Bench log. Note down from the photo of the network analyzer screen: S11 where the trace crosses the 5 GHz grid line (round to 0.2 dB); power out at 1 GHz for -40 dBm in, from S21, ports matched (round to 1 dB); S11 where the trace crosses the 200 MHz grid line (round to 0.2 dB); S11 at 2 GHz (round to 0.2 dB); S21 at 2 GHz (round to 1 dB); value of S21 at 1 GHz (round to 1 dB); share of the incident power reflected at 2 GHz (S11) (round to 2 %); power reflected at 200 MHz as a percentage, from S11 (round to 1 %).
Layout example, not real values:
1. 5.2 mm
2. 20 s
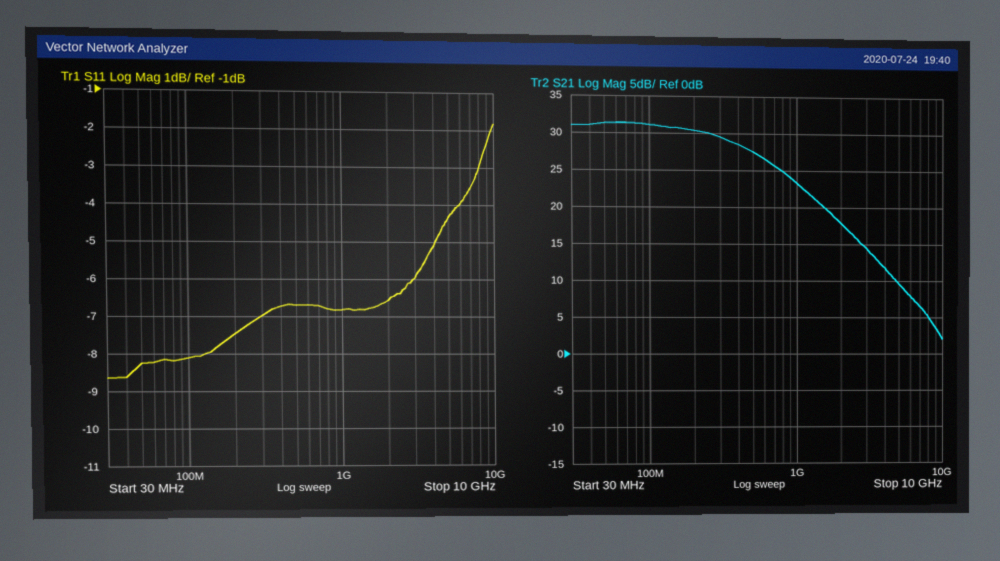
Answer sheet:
1. -4.4 dB
2. -17 dBm
3. -7.4 dB
4. -6.6 dB
5. 18 dB
6. 23 dB
7. 22 %
8. 18 %
